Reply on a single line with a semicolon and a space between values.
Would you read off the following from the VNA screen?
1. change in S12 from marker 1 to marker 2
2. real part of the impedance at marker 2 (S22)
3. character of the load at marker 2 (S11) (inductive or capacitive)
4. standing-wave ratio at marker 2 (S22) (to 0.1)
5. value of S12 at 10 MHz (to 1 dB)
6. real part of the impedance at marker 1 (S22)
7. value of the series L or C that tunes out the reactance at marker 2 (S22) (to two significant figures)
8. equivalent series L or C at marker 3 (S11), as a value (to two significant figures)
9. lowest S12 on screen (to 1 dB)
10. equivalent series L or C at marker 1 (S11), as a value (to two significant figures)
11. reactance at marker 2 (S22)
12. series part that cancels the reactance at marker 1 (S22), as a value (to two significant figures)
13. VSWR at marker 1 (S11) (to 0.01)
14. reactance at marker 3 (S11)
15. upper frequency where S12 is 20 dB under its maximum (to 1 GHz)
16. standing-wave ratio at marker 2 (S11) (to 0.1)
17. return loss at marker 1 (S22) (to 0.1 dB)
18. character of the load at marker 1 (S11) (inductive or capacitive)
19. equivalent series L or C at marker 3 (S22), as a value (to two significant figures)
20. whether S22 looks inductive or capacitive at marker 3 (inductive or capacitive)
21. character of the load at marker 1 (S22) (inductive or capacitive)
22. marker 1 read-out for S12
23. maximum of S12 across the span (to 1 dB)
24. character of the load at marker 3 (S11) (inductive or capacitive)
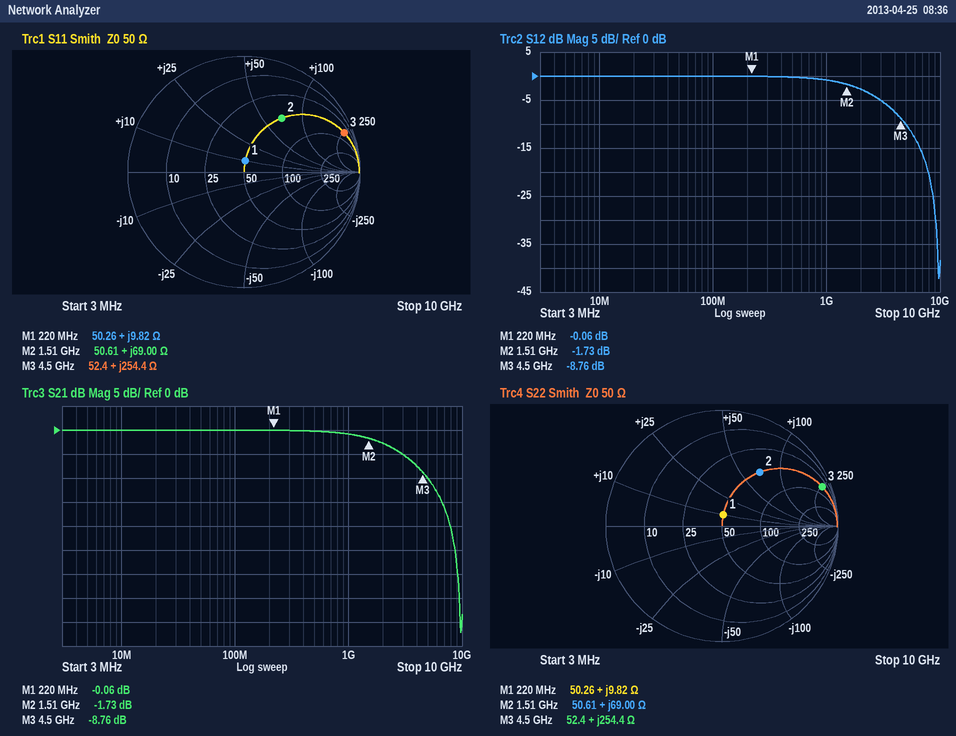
-1.67 dB; 50.61 Ω; inductive; 3.6; 0 dB; 50.26 Ω; 1.5 pF; 9.0 nH; -42 dB; 7.1 nH; +69.00 Ω; 74 pF; 1.22; +254.4 Ω; 8 GHz; 3.6; 20.2 dB; inductive; 9.0 nH; inductive; inductive; -0.06 dB; 0 dB; inductive
